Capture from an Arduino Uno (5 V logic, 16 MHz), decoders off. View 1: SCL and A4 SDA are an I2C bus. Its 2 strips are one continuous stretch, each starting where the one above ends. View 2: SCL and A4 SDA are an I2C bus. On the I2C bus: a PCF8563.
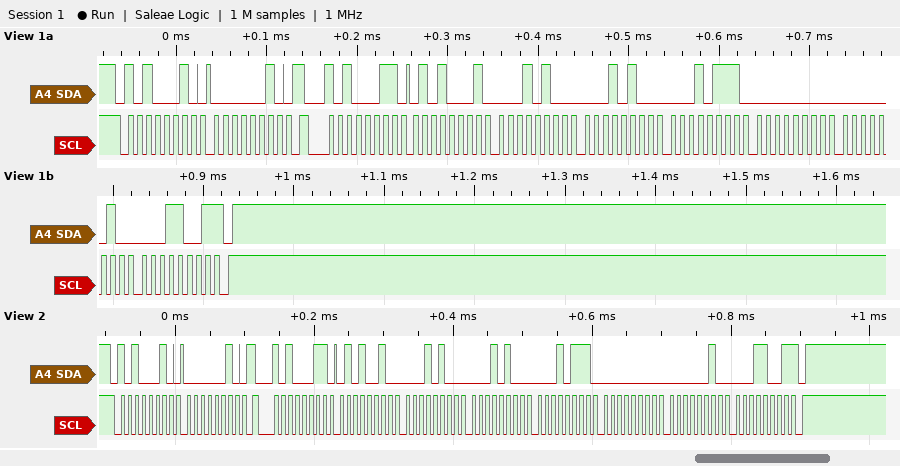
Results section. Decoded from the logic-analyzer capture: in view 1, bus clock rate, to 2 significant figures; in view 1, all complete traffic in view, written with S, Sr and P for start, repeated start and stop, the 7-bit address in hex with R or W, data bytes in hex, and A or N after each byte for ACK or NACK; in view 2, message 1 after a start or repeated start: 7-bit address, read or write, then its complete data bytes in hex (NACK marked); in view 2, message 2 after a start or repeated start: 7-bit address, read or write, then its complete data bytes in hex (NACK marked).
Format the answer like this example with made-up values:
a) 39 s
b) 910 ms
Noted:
a) 100 kHz
b) S 51W A 02 A Sr 51R A 51 A 14 A 14 A 17 A 00 A 02 A 19 N P
c) 0x51 write: 02
d) 0x51 read: 52 14 14 17 00 02 19 NACK
